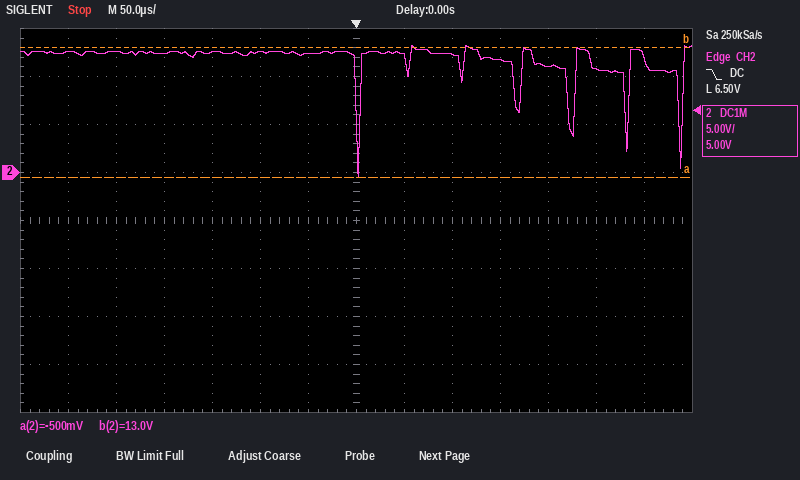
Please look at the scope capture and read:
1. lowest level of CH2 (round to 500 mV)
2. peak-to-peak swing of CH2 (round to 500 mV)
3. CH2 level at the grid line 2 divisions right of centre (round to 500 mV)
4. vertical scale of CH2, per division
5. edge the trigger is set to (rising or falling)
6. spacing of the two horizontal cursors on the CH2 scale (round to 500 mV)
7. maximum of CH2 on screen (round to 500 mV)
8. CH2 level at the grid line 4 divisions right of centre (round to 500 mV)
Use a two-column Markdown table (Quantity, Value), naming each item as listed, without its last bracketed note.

| Quantity | Value |
|---|---|
| lowest level of CH2 | -500 mV |
| peak-to-peak swing of CH2 | 13.5 V |
| CH2 level at the grid line 2 divisions right of centre | 12.5 V |
| vertical scale of CH2, per division | 5 V |
| edge the trigger is set to | falling |
| spacing of the two horizontal cursors on the CH2 scale | 13.5 V |
| maximum of CH2 on screen | 13.0 V |
| CH2 level at the grid line 4 divisions right of centre | 11.0 V |
